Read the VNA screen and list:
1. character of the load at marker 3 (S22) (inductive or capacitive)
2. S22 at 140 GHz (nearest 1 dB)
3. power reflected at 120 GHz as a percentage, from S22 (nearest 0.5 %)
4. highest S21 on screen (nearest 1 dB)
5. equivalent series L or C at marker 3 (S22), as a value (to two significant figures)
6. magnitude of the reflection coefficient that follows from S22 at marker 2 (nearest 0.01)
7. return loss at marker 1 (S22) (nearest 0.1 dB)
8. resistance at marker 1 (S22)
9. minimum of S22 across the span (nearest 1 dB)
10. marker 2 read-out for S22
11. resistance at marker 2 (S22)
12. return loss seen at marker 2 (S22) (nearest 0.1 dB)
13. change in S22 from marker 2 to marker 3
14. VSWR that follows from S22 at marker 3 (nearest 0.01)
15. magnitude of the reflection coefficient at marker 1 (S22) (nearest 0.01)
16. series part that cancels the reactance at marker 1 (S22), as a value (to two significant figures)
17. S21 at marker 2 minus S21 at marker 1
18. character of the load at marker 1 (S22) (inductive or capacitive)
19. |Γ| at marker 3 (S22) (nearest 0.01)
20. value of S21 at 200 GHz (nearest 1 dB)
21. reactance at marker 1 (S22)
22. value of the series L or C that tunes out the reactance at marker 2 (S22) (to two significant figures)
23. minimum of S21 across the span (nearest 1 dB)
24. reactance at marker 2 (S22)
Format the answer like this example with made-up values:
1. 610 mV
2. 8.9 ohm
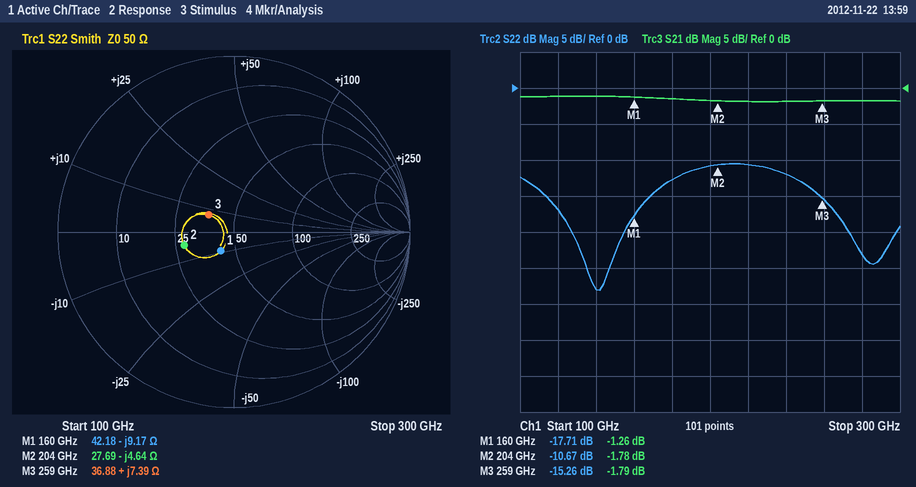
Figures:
1. inductive
2. -28 dB
3. 2.0 %
4. -1 dB
5. 4.5 pH
6. 0.29
7. 17.7 dB
8. 42.18 Ω
9. -28 dB
10. -10.67 dB
11. 27.69 Ω
12. 10.7 dB
13. -4.59 dB
14. 1.42
15. 0.13
16. 9.1 pH
17. -0.52 dB
18. capacitive
19. 0.17
20. -2 dB
21. -9.17 Ω
22. 3.6 pH
23. -2 dB
24. -4.64 Ω
